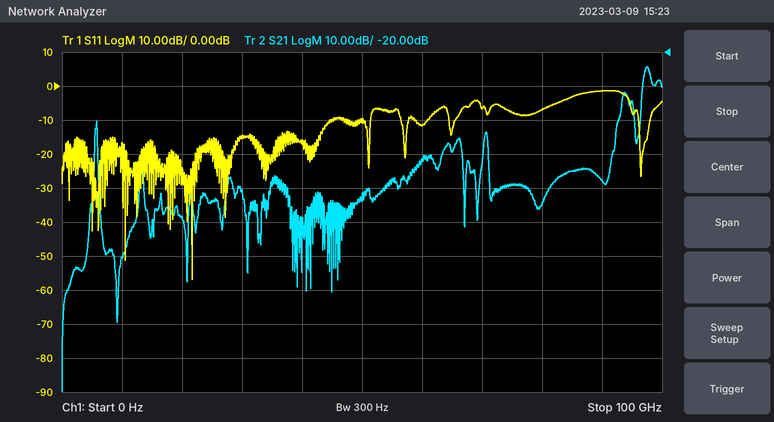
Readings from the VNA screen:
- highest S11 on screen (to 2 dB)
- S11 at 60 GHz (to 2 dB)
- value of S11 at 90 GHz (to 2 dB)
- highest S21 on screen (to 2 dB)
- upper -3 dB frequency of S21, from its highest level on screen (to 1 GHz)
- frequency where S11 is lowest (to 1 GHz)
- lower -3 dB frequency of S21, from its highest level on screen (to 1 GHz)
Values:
-2 dB
-12 dB
-2 dB
-24 dB
98 GHz
22 GHz
97 GHz
